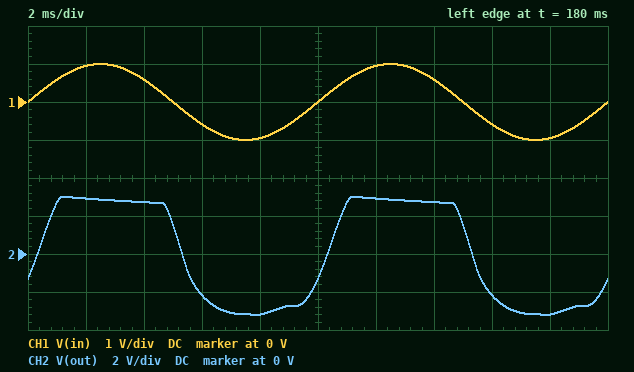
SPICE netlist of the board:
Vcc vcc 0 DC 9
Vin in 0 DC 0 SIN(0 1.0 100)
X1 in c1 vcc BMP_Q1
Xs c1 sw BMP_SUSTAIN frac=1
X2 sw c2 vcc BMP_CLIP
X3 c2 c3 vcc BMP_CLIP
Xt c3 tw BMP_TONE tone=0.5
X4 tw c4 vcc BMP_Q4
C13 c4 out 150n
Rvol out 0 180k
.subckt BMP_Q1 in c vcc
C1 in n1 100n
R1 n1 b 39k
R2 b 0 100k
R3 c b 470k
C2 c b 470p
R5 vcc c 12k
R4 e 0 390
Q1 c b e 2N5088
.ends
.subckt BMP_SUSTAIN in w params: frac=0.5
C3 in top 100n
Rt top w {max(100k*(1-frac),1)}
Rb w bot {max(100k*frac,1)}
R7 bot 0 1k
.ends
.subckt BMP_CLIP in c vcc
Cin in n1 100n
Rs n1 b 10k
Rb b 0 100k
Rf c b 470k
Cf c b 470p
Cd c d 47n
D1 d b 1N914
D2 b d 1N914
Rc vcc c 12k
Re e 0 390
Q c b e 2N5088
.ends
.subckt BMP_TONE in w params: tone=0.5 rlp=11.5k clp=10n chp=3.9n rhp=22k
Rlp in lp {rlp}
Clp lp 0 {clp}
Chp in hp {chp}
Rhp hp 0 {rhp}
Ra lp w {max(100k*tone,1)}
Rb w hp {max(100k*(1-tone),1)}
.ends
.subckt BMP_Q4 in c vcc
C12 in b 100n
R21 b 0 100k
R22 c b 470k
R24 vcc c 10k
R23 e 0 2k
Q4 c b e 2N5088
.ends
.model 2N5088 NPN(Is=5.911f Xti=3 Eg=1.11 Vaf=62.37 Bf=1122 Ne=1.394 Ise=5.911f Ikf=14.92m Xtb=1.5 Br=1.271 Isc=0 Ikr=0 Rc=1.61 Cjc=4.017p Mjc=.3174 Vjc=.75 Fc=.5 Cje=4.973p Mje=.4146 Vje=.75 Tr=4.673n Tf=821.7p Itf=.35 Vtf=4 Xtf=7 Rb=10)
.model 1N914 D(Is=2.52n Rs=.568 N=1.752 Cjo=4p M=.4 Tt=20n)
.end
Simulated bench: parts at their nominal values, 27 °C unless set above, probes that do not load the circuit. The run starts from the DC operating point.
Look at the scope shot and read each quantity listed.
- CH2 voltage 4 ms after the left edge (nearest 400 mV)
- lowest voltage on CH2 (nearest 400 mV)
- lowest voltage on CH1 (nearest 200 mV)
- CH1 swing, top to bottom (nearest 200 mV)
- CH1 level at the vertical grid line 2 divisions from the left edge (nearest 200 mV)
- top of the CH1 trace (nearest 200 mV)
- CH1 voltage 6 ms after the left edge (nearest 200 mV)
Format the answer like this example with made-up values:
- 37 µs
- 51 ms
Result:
- 2.8 V
- -3.2 V
- -1.0 V
- 2.0 V
- 600 mV
- 1.0 V
- -600 mV
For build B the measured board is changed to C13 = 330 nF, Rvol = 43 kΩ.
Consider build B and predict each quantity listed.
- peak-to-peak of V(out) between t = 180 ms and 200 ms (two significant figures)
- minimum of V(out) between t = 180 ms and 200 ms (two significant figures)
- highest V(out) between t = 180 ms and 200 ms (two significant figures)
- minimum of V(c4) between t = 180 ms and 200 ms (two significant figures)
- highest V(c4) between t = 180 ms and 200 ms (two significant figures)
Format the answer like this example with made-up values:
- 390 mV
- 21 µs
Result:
- 5.5 V
- -2.8 V
- 2.7 V
- 3.0 V
- 8.3 V
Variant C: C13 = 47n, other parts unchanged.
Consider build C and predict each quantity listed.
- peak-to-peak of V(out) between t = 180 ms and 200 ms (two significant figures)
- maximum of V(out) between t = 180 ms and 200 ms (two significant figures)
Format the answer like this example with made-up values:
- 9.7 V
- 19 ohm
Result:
- 6.5 V
- 3.3 V
